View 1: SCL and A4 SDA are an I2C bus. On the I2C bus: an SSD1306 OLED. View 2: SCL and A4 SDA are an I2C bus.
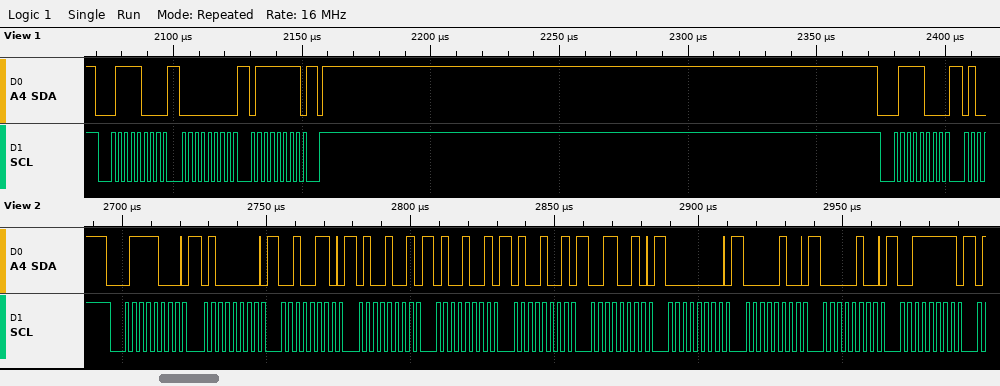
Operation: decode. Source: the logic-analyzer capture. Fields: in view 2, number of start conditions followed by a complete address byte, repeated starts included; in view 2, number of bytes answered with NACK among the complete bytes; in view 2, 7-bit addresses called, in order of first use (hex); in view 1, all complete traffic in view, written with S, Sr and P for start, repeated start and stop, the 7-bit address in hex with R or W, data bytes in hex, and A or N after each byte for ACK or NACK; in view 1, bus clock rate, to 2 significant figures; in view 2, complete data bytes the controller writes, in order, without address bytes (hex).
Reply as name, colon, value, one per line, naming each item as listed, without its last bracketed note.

in view 2, number of start conditions followed by a complete address byte, repeated starts included: 1
in view 2, number of bytes answered with NACK among the complete bytes: 0
in view 2, 7-bit addresses called, in order of first use: 0x3C
in view 1, all complete traffic in view, written with S, Sr and P for start, repeated start and stop, the 7-bit address in hex with R or W, data bytes in hex, and A or N after each byte for ACK or NACK: S 3CW A 00 A 7F A P S 3CW A
in view 1, bus clock rate, to 2 significant figures: 400 kHz
in view 2, complete data bytes the controller writes, in order, without address bytes: 40 26 49 49 49 32 00 04 04 3F
